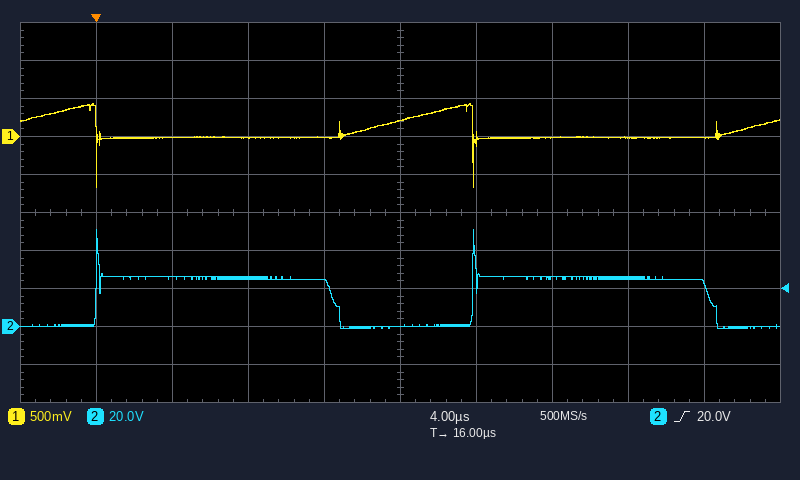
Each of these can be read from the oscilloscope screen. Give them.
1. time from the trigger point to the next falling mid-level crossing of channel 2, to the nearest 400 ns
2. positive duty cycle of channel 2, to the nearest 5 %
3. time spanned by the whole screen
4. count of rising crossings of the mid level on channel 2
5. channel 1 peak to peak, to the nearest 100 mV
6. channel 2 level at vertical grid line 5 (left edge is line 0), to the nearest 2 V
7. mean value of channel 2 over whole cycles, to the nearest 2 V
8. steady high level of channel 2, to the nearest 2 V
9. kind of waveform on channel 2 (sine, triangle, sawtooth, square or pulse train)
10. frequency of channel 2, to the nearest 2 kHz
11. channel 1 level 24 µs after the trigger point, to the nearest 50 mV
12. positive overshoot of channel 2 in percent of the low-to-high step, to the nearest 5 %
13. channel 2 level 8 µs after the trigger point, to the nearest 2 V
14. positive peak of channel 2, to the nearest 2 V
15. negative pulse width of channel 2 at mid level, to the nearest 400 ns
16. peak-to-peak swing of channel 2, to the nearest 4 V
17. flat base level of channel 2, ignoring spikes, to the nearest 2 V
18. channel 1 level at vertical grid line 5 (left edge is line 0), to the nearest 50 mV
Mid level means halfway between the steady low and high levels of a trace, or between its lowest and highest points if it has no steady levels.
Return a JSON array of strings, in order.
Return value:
["12.4 µs", "65 %", "40 µs", "2", "1.10 V", "0 V", "16 V", "26 V", "pulse train", "50 kHz", "0 mV", "100 %", "26 V", "52 V", "7.2 µs", "52 V", "0 V", "200 mV"]
